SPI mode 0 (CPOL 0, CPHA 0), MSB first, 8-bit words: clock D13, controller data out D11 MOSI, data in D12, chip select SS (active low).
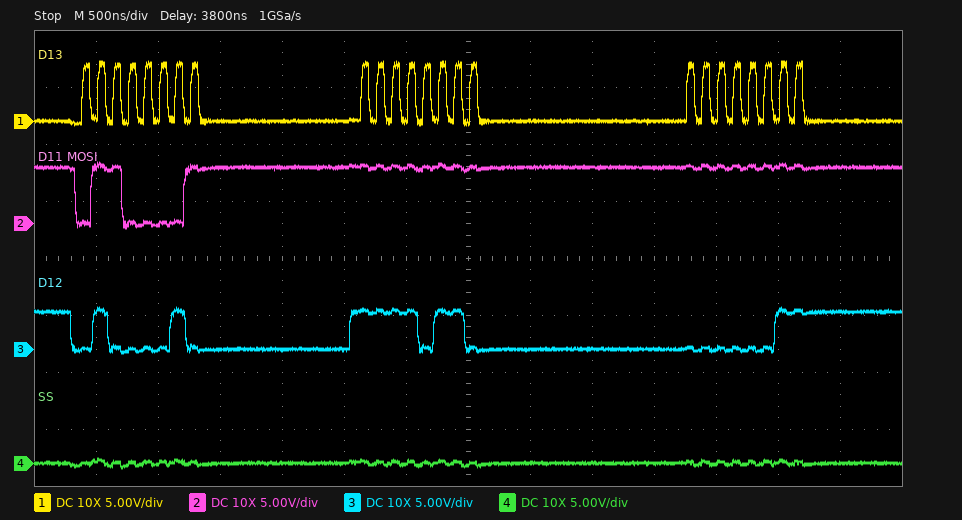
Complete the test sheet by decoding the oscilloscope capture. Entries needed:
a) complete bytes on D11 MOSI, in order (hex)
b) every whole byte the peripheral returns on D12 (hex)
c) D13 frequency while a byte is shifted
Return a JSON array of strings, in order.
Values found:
["61 FF FF", "42 F6 03", "8 MHz"]
